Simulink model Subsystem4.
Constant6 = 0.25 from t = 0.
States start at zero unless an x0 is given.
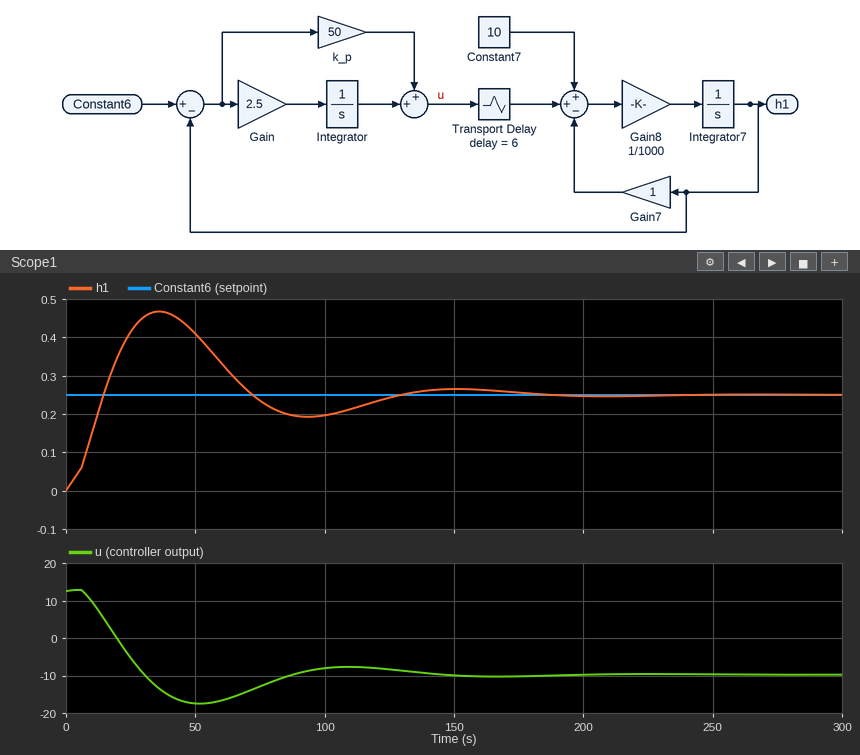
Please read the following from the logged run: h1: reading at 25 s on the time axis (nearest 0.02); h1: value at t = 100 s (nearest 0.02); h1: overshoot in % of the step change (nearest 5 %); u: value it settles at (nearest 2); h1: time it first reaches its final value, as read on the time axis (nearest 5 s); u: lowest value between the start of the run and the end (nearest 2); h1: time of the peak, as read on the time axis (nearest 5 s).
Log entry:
0.42
0.20
85 %
-10
15 s
-18
35 s
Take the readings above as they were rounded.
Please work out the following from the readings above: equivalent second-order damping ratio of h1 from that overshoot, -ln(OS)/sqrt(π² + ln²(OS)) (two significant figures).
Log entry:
0.052
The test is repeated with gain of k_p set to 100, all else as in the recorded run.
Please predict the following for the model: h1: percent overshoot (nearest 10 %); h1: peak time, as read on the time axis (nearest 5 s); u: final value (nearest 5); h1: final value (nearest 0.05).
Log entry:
70 %
25 s
-10
0.25
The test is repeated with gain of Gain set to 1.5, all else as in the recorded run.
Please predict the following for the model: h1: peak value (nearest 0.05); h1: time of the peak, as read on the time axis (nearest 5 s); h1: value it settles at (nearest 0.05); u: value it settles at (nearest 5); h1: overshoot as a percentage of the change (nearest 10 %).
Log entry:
0.45
40 s
0.25
-10
80 %
